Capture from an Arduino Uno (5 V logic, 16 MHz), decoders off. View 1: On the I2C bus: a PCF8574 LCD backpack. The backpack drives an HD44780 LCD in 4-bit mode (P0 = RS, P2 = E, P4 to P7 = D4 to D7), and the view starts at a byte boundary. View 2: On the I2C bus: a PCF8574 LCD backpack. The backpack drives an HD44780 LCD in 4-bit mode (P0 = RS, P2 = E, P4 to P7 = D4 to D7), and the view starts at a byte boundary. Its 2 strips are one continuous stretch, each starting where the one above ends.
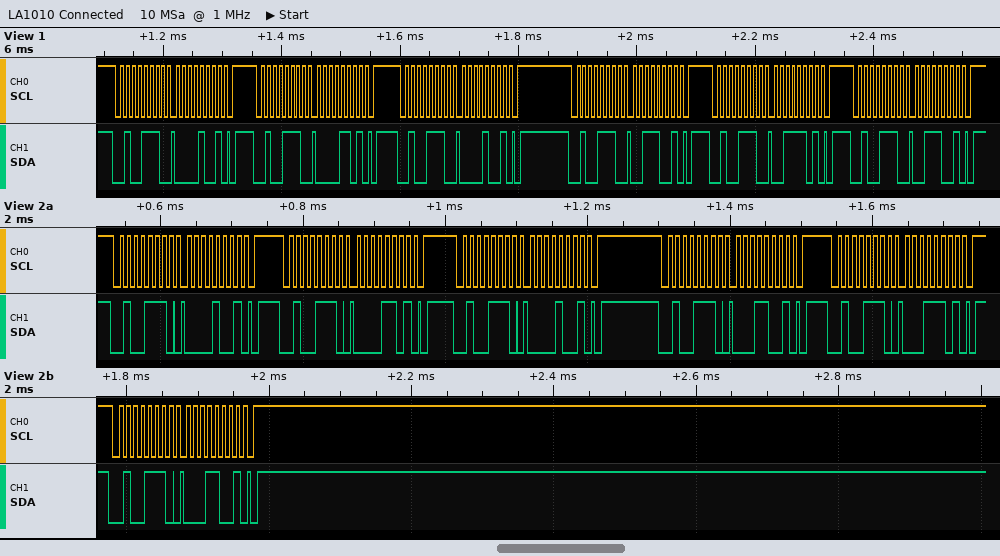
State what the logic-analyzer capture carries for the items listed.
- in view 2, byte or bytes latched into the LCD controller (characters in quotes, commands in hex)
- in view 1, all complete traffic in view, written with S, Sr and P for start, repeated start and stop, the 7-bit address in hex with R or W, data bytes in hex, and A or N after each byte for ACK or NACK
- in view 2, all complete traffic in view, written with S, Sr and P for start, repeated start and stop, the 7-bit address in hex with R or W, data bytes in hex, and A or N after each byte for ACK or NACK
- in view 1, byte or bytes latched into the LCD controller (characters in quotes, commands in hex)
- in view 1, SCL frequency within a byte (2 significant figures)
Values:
data 0x01
S 27W A 09 A P S 27W A 0D A P S 27W A 09 A P S 27W A 39 A P S 27W A 3D A P S 27W A 39 A P
S 27W A 09 A P S 27W A 0D A P S 27W A 09 A P S 27W A 19 A P S 27W A 1D A P S 27W A 19 A P
data 0x03
100 kHz
